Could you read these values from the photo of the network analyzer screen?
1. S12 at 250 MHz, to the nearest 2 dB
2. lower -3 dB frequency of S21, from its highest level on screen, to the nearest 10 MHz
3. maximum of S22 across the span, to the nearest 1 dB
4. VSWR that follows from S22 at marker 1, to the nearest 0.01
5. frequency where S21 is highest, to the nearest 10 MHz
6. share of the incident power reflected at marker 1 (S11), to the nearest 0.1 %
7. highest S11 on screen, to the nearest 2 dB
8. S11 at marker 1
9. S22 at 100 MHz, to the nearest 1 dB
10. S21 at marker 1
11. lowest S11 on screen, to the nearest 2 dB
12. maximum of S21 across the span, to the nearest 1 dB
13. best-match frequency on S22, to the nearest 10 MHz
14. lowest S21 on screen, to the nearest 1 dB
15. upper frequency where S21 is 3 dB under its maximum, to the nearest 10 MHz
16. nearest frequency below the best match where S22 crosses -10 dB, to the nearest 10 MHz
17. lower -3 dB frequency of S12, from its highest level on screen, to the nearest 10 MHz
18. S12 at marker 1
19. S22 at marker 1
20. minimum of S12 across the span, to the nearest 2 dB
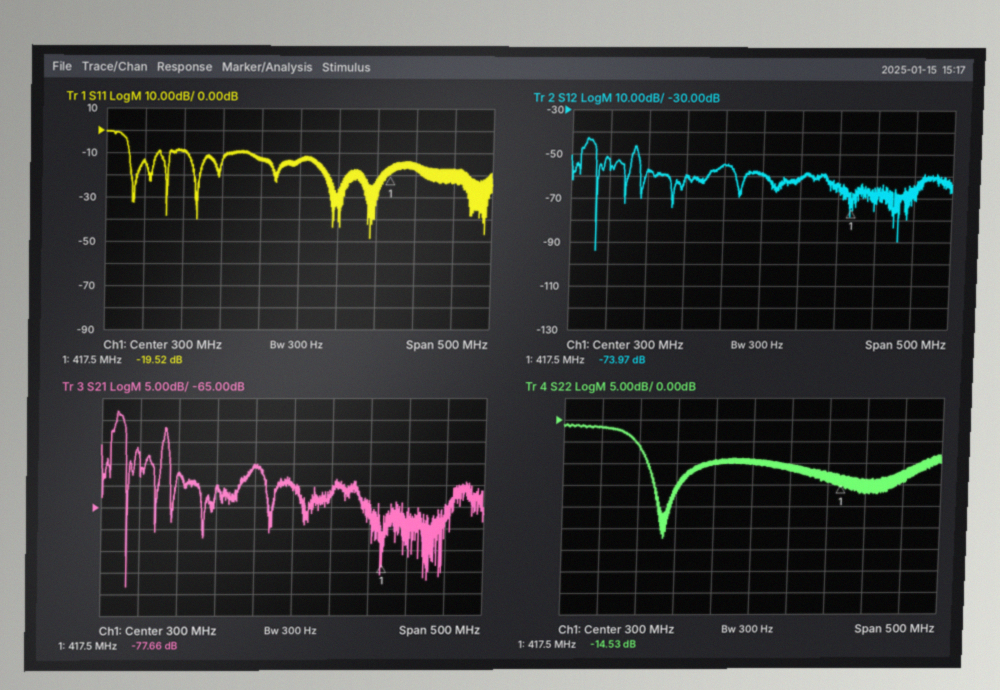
-54 dB
70 MHz
-1 dB
1.46
70 MHz
1.1 %
0 dB
-19.52 dB
-2 dB
-77.66 dB
-48 dB
-43 dB
180 MHz
-83 dB
80 MHz
160 MHz
70 MHz
-73.97 dB
-14.53 dB
-94 dB
